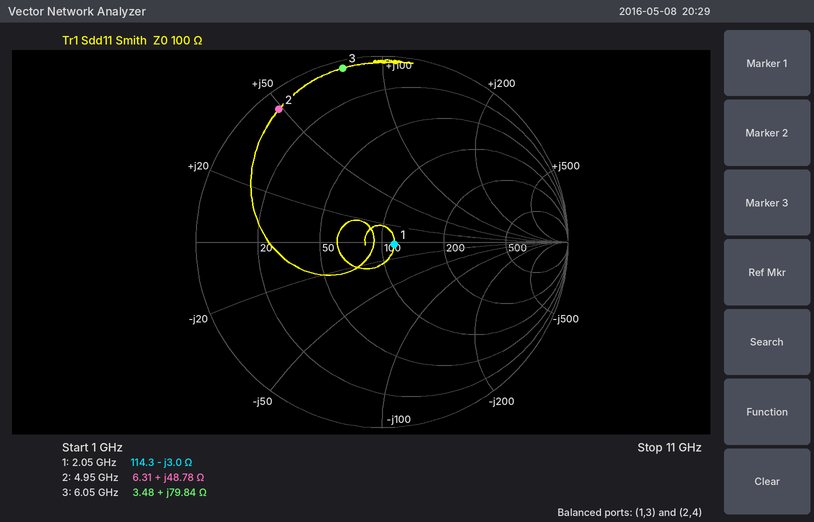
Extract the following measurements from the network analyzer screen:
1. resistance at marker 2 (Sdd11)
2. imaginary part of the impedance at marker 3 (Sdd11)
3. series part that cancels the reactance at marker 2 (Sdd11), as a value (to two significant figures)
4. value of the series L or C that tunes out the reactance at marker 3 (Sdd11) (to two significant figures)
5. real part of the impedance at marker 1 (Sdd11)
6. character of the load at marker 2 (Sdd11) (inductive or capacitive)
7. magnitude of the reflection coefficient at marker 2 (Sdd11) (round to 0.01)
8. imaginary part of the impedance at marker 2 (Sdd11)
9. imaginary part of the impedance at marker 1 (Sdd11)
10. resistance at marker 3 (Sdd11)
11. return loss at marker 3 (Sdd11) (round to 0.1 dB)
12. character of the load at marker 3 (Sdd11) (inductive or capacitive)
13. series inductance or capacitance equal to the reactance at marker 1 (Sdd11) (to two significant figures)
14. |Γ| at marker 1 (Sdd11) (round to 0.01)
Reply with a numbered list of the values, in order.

1. 6.31 Ω
2. +79.84 Ω
3. 660 fF
4. 330 fF
5. 114.3 Ω
6. inductive
7. 0.90
8. +48.78 Ω
9. -3.0 Ω
10. 3.48 Ω
11. 0.4 dB
12. inductive
13. 26 pF
14. 0.07
